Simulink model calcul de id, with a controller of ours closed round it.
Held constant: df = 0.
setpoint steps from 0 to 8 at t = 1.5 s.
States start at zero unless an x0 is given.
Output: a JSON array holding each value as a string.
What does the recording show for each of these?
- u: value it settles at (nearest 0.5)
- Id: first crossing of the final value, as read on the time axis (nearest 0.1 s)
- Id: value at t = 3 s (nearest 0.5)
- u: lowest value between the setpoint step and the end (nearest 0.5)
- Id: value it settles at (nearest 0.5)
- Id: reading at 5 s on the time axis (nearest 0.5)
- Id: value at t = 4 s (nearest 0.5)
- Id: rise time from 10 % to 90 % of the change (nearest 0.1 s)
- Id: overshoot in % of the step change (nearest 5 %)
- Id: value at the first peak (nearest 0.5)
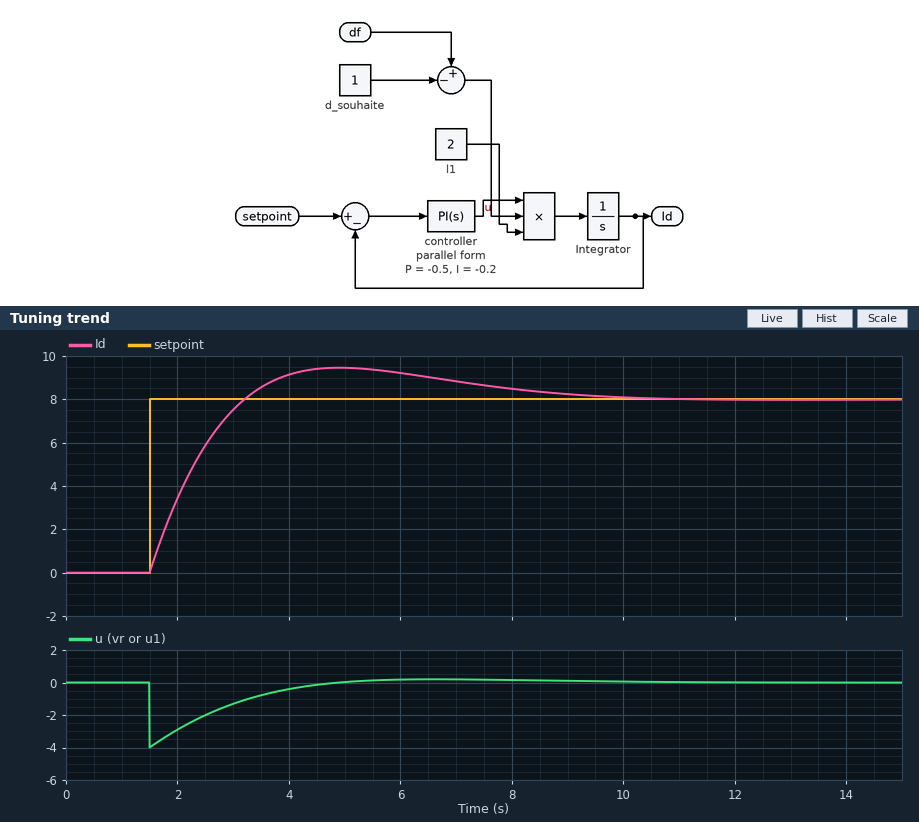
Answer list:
["0.0", "3.2 s", "7.5", "-4.0", "8.0", "9.5", "9.0", "1.3 s", "20 %", "9.5"]
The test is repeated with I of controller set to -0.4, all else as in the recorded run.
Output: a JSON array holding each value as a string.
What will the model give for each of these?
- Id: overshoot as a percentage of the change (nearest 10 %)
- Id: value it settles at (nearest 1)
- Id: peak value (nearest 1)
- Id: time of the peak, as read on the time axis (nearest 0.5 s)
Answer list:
["30 %", "8", "10", "4.0 s"]
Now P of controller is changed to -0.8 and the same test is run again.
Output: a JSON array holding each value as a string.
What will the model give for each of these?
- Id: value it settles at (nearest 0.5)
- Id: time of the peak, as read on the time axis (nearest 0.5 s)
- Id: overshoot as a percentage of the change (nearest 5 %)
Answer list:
["8.0", "4.5 s", "10 %"]
